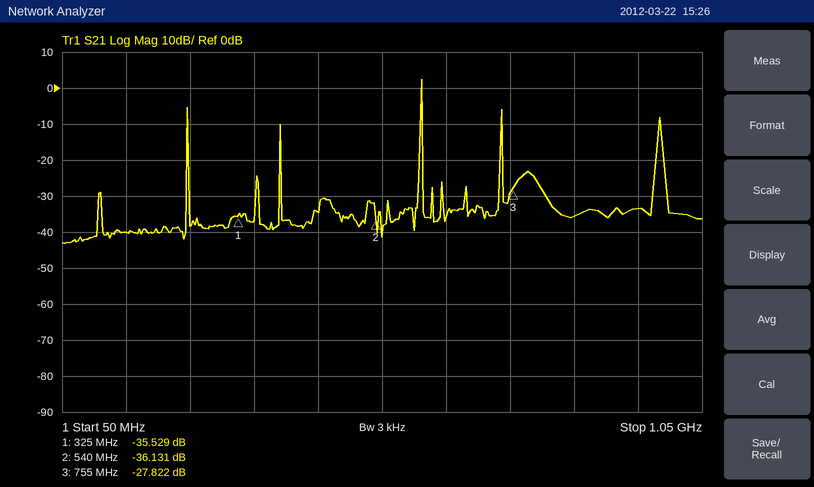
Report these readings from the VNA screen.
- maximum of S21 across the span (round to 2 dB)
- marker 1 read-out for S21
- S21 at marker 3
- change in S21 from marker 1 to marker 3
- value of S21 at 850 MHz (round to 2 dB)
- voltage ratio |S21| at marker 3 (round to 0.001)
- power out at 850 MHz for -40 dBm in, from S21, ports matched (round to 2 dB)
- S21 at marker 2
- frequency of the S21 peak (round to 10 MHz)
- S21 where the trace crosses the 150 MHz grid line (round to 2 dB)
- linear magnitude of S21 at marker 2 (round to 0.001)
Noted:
2 dB
-35.529 dB
-27.822 dB
7.707 dB
-36 dB
0.041
-76 dBm
-36.131 dB
610 MHz
-40 dB
0.016
